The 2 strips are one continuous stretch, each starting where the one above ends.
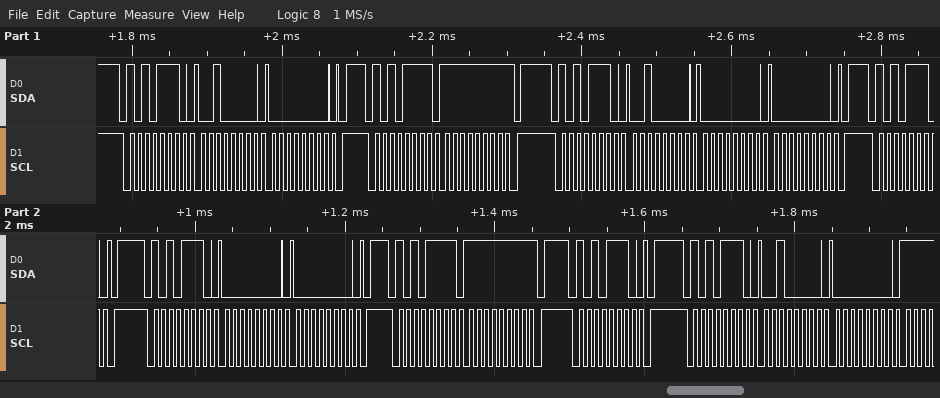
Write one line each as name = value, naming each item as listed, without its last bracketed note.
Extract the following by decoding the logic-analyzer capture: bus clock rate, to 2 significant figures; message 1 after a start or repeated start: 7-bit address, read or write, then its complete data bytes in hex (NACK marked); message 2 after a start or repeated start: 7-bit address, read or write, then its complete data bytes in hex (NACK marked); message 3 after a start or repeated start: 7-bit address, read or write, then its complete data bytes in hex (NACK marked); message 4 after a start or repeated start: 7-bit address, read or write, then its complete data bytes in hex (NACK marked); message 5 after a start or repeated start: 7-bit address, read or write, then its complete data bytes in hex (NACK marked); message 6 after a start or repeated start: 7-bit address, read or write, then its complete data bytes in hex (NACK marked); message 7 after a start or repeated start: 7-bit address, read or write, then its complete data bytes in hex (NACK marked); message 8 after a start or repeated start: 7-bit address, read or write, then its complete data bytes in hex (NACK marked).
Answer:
bus clock rate, to 2 significant figures = 100 kHz
message 1 after a start or repeated start: 7-bit address, read or write, then its complete data bytes in hex = 0x57 write: 20 00
message 2 after a start or repeated start: 7-bit address, read or write, then its complete data bytes in hex = 0x57 read: FF NACK
message 3 after a start or repeated start: 7-bit address, read or write, then its complete data bytes in hex = 0x57 write: 20 00 00
message 4 after a start or repeated start: 7-bit address, read or write, then its complete data bytes in hex = 0x57 write
message 5 after a start or repeated start: 7-bit address, read or write, then its complete data bytes in hex = 0x57 write: 00 00
message 6 after a start or repeated start: 7-bit address, read or write, then its complete data bytes in hex = 0x57 read: FF NACK
message 7 after a start or repeated start: 7-bit address, read or write, then its complete data bytes in hex = 0x57 write
message 8 after a start or repeated start: 7-bit address, read or write, then its complete data bytes in hex = 0x57 write: 20 00
